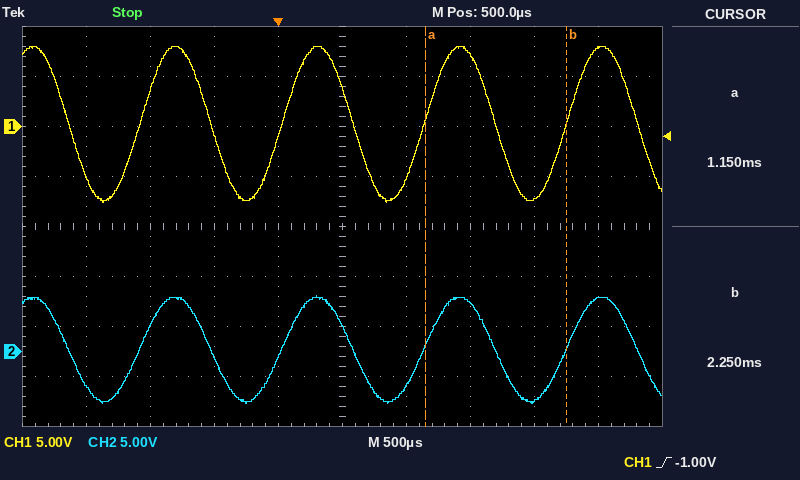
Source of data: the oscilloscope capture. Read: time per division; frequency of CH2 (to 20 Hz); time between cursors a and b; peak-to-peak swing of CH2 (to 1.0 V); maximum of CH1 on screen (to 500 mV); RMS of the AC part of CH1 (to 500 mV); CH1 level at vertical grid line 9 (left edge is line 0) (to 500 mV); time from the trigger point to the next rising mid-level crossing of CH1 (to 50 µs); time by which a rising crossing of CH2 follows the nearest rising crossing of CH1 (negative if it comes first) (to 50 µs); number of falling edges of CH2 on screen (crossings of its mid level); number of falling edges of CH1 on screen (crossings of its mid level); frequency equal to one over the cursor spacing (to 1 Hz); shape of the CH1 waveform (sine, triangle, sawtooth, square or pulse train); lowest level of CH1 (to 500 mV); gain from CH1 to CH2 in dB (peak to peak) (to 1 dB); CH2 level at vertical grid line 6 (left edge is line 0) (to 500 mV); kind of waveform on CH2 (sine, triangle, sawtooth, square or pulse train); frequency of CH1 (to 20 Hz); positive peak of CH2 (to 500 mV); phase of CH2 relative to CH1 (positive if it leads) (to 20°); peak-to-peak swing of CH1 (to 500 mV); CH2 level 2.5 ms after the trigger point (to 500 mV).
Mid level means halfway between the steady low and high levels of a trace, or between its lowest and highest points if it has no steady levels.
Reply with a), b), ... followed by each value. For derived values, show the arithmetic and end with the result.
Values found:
a) 500 µs
b) 900 Hz
c) 2.25 ms − (1.15 ms) = 1.10 ms
d) 11.0 V
e) 8.0 V
f) 15.5 V / (2√2) ≈ 5.5 V
g) 8.0 V
h) 50 µs
i) 0 µs
j) 5
k) 5
l) 1 / 1.10 ms ≈ 909 Hz
m) sine
n) -7.5 V
o) 20 log10(11.0 V / 15.5 V) ≈ -3 dB
p) -3.5 V
q) sine
r) 900 Hz
s) 5.5 V
t) 0°
u) 8.0 V − (-7.5 V) = 15.5 V
v) 5.5 V
